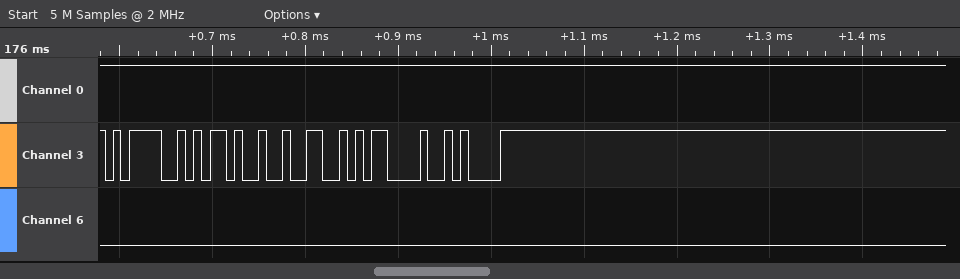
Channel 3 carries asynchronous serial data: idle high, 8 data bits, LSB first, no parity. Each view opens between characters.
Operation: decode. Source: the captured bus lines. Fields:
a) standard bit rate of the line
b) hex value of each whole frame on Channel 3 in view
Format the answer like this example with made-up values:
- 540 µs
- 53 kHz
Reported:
- 115200 baud
- 3D, 2D, 32, 0D, 0A
